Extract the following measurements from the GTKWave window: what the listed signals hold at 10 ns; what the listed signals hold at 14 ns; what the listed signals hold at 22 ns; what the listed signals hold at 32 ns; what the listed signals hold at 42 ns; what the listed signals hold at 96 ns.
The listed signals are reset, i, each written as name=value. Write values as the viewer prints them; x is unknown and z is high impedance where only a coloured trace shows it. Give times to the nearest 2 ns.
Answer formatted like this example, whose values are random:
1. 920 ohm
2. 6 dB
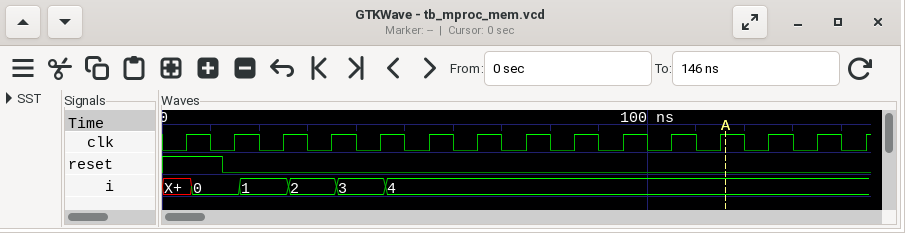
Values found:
1. reset=1, i=0
2. reset=0, i=0
3. reset=0, i=1
4. reset=0, i=2
5. reset=0, i=3
6. reset=0, i=4
